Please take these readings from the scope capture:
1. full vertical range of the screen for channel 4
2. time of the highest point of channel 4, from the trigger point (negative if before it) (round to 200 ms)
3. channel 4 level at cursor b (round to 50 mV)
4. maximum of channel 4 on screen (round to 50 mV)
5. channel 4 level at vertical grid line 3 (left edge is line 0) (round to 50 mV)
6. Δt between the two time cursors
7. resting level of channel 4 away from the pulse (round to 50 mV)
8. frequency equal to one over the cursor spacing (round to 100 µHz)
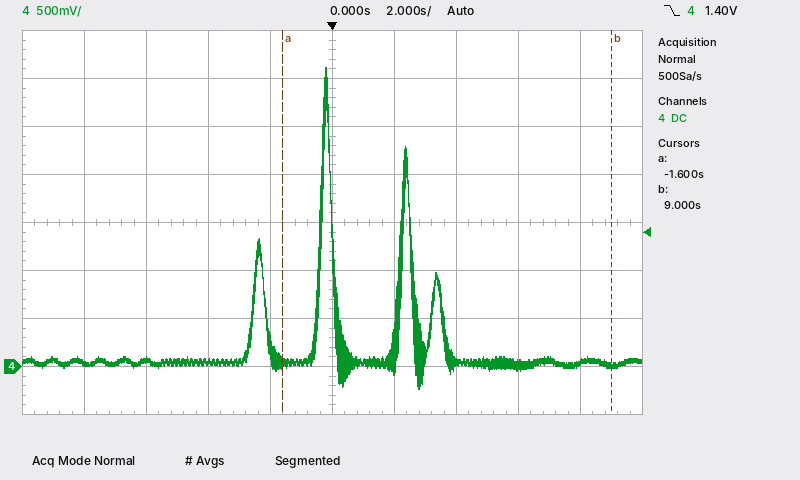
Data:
4 V
-200 ms
0 mV
3.10 V
50 mV
10.6 s
50 mV
94.3 mHz
